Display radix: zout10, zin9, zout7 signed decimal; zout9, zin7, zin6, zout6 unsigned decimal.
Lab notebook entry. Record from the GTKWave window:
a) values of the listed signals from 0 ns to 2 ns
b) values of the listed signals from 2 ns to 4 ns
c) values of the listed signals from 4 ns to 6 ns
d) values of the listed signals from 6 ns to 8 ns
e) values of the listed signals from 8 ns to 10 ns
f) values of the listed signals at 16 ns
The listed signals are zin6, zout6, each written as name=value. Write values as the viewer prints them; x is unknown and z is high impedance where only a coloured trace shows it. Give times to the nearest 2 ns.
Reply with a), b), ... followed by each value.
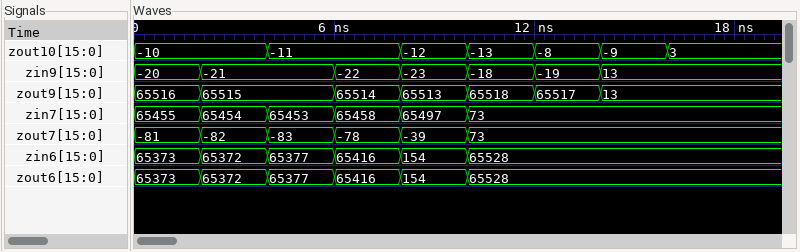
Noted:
a) zin6=65373, zout6=65373
b) zin6=65372, zout6=65372
c) zin6=65377, zout6=65377
d) zin6=65416, zout6=65416
e) zin6=154, zout6=154
f) zin6=65528, zout6=65528
